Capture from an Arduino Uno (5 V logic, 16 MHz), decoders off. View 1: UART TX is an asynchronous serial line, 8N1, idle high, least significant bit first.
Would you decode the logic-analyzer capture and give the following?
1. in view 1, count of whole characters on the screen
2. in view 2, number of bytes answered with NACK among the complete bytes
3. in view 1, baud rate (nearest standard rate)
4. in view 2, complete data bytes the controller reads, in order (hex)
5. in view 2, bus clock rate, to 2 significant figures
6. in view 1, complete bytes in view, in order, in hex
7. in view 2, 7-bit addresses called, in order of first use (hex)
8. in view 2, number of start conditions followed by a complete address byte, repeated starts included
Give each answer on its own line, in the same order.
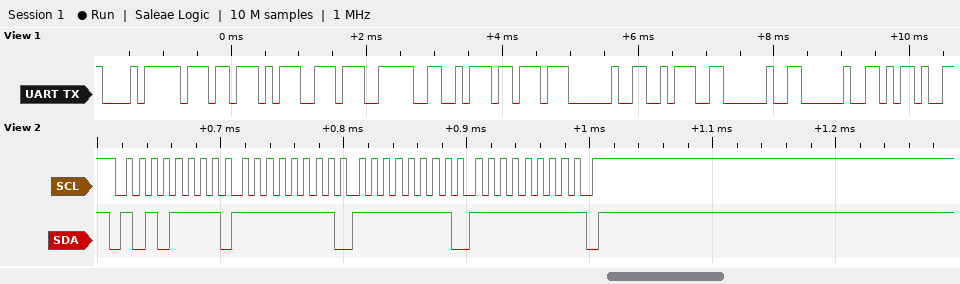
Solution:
11
1
9600 baud
FF FF FF
100 kHz
E8 B7 9D E7 A6 BB 20 3A 20 20 2D
0x57
1
